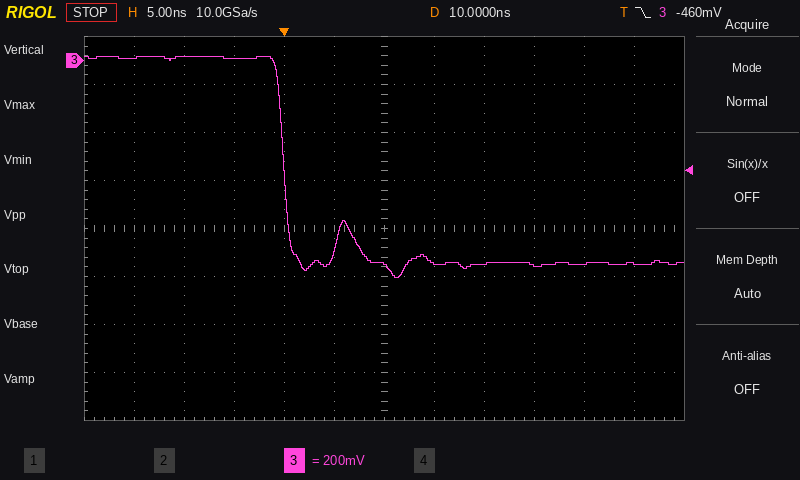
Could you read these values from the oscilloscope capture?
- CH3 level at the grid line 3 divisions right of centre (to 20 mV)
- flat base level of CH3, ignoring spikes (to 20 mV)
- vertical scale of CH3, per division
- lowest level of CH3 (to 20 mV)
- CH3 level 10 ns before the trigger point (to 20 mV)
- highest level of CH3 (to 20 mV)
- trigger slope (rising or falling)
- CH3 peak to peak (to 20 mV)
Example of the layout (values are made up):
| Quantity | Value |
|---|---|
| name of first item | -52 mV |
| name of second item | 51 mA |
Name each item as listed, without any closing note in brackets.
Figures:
| Quantity | Value |
|---|---|
| CH3 level at the grid line 3 divisions right of centre | -860 mV |
| flat base level of CH3, ignoring spikes | -840 mV |
| vertical scale of CH3, per division | 200 mV |
| lowest level of CH3 | -900 mV |
| CH3 level 10 ns before the trigger point | 20 mV |
| highest level of CH3 | 20 mV |
| trigger slope | falling |
| CH3 peak to peak | 920 mV |
